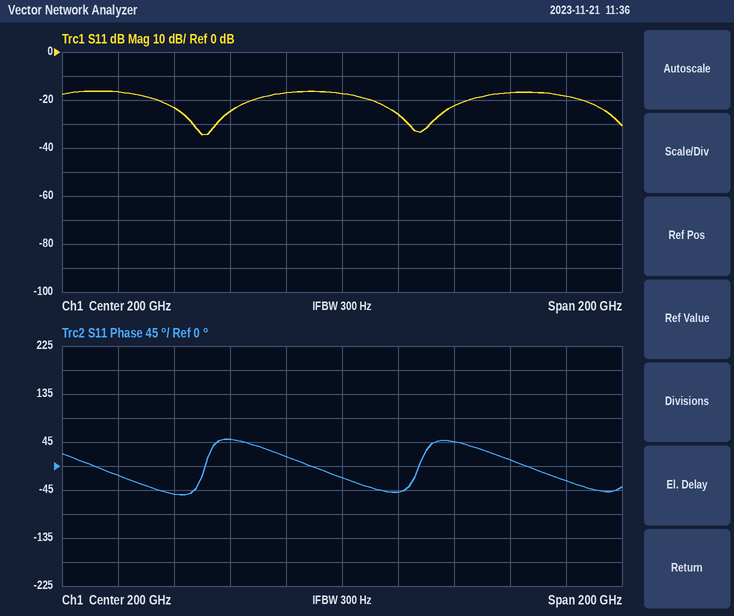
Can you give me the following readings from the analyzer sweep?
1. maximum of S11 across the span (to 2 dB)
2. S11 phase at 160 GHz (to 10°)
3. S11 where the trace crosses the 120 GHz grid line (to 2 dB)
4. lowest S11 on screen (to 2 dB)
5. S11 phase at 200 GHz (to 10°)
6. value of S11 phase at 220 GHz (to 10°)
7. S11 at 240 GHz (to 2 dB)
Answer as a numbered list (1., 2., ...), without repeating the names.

1. -16 dB
2. 50°
3. -16 dB
4. -34 dB
5. -20°
6. -50°
7. -22 dB
